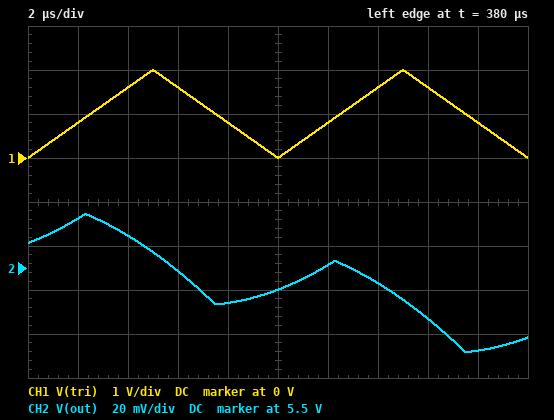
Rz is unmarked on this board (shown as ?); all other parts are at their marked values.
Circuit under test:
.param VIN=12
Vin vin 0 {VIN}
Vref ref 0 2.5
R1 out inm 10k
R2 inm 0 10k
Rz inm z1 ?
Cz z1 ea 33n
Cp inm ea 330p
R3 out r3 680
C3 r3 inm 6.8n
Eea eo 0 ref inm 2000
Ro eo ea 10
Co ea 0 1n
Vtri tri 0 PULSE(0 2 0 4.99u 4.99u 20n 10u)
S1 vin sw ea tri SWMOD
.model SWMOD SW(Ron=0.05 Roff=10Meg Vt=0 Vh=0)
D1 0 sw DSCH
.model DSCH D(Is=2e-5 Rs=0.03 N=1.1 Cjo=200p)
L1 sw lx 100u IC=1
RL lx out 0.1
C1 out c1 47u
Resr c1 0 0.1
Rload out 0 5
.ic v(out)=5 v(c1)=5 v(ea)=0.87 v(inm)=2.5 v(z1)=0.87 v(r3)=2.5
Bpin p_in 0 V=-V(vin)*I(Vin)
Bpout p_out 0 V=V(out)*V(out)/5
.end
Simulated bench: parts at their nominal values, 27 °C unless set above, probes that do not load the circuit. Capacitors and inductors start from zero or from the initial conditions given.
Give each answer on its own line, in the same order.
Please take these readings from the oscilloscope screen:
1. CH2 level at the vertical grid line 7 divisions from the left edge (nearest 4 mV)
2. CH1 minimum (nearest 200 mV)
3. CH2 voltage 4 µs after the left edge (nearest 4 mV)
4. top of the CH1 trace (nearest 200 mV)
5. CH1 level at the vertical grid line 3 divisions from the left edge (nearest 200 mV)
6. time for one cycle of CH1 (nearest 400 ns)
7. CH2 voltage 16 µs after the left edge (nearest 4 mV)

5.492 V
0 V
5.516 V
2.0 V
1.6 V
10.0 µs
5.476 V
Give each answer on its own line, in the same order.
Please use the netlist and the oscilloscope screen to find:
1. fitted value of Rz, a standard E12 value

3.3 kΩ
